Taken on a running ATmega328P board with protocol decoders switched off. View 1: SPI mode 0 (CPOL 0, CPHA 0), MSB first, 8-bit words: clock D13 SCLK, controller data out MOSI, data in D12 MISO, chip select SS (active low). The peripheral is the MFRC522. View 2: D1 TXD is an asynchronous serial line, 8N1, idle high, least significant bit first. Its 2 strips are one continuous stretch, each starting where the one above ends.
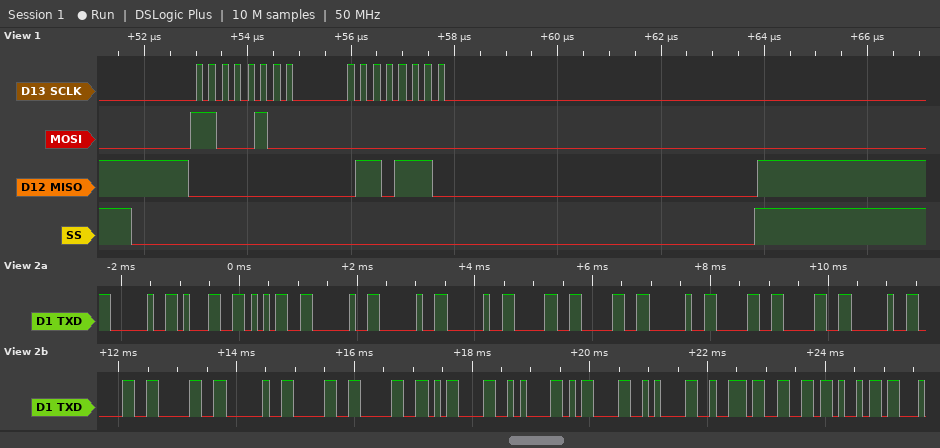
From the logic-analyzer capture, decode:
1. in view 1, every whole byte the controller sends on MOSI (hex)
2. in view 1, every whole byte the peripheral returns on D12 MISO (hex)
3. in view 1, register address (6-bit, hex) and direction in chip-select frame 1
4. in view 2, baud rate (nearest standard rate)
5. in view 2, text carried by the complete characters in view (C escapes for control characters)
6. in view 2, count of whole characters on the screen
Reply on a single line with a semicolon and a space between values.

C4 00; 00 6E; 0x22 read; 9600 baud; " 15   00 00 00 00\r\n\r\nrfi"; 24
